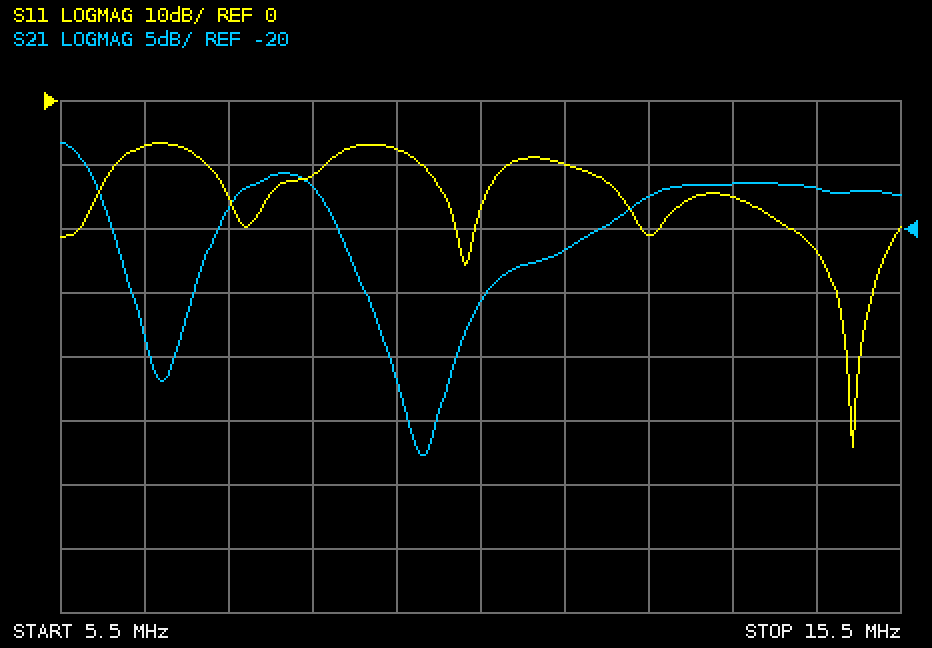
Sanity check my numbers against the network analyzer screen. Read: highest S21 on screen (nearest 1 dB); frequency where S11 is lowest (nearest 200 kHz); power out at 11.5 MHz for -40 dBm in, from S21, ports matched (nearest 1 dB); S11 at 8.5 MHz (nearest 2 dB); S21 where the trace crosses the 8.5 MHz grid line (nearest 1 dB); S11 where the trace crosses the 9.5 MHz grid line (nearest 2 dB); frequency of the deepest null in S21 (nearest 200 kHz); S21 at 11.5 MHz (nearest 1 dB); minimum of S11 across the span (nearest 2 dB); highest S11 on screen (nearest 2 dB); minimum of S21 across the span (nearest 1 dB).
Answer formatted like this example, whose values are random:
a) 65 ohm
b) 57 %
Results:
a) -13 dB
b) 15.0 MHz
c) -62 dBm
d) -12 dB
e) -17 dB
f) -8 dB
g) 9.8 MHz
h) -22 dB
i) -54 dB
j) -6 dB
k) -38 dB
